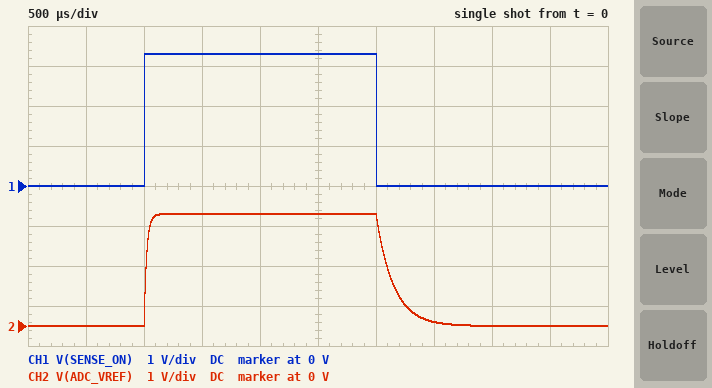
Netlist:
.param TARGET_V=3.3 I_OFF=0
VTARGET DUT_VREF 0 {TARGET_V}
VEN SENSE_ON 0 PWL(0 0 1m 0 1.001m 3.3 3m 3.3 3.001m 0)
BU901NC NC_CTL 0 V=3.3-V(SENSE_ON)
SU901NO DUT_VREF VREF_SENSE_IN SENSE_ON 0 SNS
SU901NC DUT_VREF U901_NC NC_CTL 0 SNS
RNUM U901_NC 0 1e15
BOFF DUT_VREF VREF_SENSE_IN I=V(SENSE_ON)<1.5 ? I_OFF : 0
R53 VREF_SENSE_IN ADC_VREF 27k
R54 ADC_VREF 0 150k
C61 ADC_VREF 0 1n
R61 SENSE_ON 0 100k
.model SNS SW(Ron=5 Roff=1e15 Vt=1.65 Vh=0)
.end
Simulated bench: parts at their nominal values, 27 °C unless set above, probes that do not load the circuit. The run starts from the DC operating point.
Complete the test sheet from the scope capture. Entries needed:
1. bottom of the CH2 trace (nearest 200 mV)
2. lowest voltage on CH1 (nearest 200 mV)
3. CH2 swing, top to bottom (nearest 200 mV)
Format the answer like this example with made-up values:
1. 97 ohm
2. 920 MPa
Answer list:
1. 0 V
2. 0 V
3. 2.8 V
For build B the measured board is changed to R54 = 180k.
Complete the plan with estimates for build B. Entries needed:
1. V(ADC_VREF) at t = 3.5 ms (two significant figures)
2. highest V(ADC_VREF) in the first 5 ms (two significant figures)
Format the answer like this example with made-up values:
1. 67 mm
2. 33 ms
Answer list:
1. 180 mV
2. 2.9 V
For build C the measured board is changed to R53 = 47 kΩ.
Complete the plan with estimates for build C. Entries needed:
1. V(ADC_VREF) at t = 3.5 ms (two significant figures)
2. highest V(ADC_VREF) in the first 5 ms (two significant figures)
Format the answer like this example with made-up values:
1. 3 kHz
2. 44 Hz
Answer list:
1. 90 mV
2. 2.5 V
